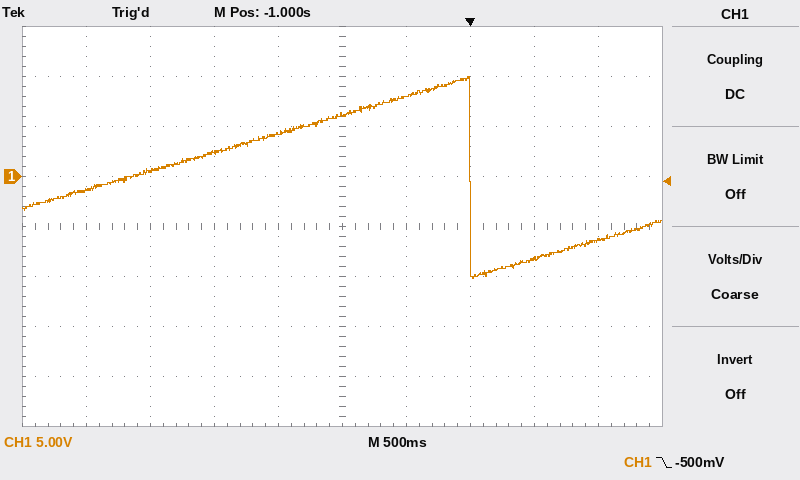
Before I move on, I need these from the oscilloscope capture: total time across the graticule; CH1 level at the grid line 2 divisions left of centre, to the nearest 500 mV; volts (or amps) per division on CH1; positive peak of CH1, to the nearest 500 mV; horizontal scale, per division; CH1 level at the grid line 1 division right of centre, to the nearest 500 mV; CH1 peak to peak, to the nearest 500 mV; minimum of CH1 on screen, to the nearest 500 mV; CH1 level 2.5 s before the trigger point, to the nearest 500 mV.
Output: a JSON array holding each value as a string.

["5 s", "2.5 V", "5 V", "10.0 V", "500 ms", "8.0 V", "20.0 V", "-10.0 V", "500 mV"]
